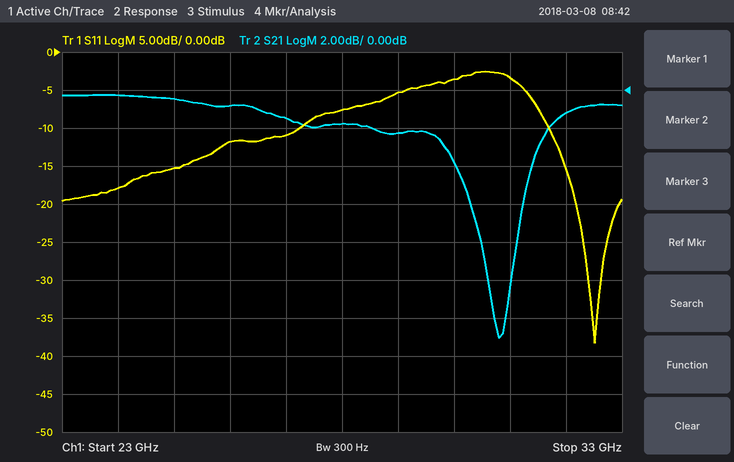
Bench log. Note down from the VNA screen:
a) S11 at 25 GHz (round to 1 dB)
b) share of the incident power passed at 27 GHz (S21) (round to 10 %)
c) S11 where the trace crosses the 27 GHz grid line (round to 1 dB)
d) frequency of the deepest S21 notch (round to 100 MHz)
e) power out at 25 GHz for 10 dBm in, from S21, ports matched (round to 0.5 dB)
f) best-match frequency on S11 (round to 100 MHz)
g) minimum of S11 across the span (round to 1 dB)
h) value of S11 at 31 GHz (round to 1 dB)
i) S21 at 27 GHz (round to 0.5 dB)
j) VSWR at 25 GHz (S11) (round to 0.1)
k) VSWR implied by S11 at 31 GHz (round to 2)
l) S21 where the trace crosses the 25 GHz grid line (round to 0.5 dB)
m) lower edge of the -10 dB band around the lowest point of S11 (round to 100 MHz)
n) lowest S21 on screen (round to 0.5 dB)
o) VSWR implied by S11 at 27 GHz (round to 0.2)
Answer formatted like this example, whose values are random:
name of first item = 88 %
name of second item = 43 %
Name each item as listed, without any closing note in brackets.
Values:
S11 at 25 GHz = -15 dB
share of the incident power passed at 27 GHz (S21) = 70 %
S11 where the trace crosses the 27 GHz grid line = -11 dB
frequency of the deepest S21 notch = 30.8 GHz
power out at 25 GHz for 10 dBm in, from S21, ports matched = 9.5 dBm
best-match frequency on S11 = 32.5 GHz
minimum of S11 across the span = -38 dB
value of S11 at 31 GHz = -3 dB
S21 at 27 GHz = -1.5 dB
VSWR at 25 GHz (S11) = 1.4
VSWR implied by S11 at 31 GHz = 6
S21 where the trace crosses the 25 GHz grid line = -0.5 dB
lower edge of the -10 dB band around the lowest point of S11 = 31.7 GHz
lowest S21 on screen = -13.0 dB
VSWR implied by S11 at 27 GHz = 1.8
